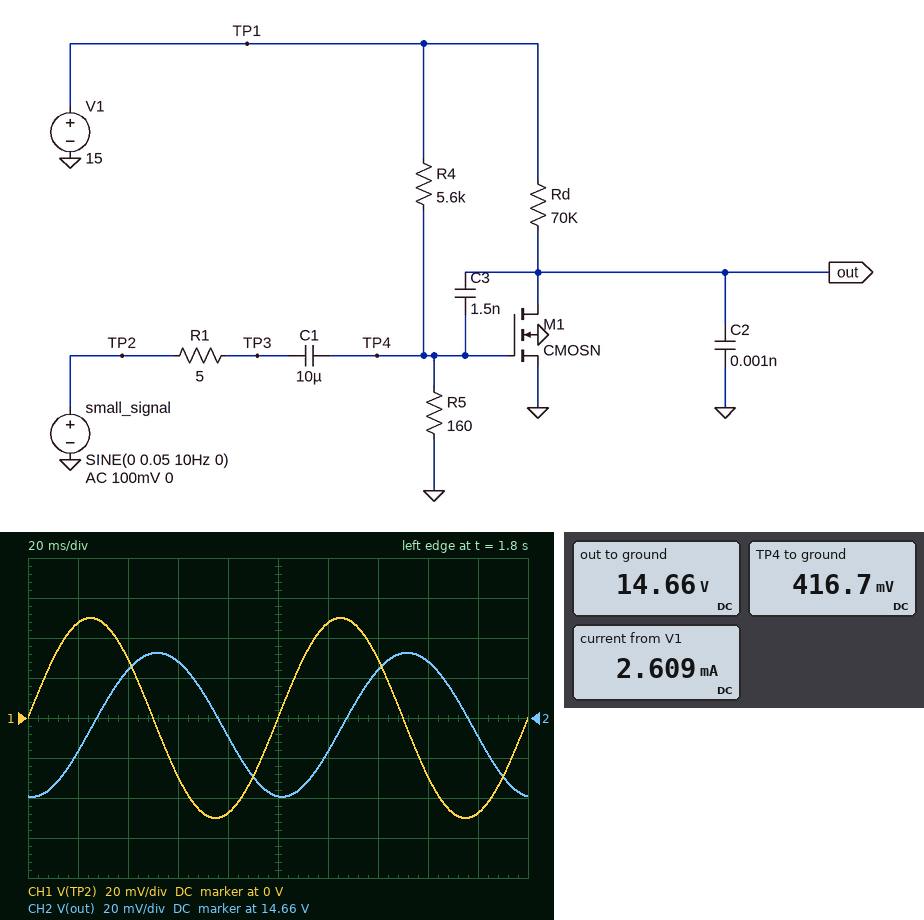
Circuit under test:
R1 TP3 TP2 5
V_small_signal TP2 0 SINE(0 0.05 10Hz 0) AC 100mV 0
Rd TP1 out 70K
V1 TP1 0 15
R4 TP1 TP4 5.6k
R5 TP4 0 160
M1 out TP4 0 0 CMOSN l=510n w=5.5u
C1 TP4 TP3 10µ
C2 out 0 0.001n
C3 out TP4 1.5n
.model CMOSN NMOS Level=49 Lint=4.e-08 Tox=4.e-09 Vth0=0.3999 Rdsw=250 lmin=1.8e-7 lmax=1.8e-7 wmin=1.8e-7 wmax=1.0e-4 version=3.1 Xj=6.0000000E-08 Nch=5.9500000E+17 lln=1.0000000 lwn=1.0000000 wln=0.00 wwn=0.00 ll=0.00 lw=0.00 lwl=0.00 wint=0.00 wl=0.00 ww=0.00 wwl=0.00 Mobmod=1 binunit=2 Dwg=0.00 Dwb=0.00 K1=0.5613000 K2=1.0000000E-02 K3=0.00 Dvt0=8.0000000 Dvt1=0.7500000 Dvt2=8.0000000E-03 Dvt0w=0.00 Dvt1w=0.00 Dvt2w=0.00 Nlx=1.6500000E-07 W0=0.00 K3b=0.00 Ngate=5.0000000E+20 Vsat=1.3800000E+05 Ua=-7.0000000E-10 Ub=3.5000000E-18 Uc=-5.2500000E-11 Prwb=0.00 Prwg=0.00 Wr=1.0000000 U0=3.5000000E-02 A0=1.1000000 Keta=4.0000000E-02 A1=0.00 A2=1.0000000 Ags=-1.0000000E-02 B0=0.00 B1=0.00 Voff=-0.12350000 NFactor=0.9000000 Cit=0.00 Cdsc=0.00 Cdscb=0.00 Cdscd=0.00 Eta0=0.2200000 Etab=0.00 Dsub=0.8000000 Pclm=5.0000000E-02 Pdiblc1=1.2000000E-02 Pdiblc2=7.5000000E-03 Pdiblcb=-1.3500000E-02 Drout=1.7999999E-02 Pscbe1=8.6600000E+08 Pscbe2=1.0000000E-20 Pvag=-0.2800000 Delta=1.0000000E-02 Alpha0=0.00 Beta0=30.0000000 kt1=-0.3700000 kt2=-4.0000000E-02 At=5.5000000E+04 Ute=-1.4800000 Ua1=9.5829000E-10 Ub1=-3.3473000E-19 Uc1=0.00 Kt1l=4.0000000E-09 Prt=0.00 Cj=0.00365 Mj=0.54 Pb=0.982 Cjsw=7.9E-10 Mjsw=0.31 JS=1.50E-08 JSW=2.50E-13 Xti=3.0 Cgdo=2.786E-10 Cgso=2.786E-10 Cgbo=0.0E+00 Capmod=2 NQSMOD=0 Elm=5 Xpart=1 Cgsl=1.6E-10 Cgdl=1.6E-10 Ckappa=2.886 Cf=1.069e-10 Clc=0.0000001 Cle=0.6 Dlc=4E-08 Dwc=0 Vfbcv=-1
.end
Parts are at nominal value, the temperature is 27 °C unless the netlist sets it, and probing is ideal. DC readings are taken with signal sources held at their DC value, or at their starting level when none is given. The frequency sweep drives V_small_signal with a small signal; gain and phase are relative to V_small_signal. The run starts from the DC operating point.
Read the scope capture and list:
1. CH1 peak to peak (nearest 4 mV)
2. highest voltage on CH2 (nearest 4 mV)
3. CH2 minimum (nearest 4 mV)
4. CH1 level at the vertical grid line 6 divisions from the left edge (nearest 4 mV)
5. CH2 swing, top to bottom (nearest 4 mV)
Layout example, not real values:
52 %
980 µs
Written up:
100 mV
14.692 V
14.620 V
48 mV
72 mV
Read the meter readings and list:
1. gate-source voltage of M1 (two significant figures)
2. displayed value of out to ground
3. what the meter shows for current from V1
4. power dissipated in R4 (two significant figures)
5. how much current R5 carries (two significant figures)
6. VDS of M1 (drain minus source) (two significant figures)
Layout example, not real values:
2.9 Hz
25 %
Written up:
420 mV
14.66 V
2.609 mA
38 mW
2.6 mA
15 V
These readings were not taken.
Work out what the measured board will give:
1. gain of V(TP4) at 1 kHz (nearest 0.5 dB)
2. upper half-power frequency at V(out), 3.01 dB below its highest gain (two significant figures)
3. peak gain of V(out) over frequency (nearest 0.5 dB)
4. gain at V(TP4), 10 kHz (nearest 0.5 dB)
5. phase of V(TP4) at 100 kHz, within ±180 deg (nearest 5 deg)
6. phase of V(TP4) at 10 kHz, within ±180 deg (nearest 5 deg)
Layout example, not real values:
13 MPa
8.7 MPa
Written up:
-0.5 dB
1.8 kHz
16.5 dB
-0.5 dB
0 deg
0 deg
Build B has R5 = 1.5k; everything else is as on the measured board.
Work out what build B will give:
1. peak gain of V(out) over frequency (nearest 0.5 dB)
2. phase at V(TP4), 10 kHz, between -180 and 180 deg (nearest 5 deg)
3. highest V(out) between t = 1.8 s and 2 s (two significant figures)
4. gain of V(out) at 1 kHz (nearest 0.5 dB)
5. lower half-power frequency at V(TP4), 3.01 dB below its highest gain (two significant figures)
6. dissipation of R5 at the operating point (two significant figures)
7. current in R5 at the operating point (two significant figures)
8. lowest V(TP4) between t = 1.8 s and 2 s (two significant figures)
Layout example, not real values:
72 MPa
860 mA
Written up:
0 dB
0 deg
80 mV
-46.5 dB
13 Hz
6.7 mW
2.1 mA
3.1 V
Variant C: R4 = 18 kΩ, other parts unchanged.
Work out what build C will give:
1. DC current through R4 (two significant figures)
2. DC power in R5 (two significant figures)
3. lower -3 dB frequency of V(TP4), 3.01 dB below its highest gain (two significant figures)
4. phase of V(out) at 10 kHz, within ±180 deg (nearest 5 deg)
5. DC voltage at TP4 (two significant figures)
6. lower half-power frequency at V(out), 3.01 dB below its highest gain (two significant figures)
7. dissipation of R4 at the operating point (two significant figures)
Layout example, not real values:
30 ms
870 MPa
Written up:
830 µA
110 µW
97 Hz
10 deg
130 mV
1.5 kHz
12 mW
